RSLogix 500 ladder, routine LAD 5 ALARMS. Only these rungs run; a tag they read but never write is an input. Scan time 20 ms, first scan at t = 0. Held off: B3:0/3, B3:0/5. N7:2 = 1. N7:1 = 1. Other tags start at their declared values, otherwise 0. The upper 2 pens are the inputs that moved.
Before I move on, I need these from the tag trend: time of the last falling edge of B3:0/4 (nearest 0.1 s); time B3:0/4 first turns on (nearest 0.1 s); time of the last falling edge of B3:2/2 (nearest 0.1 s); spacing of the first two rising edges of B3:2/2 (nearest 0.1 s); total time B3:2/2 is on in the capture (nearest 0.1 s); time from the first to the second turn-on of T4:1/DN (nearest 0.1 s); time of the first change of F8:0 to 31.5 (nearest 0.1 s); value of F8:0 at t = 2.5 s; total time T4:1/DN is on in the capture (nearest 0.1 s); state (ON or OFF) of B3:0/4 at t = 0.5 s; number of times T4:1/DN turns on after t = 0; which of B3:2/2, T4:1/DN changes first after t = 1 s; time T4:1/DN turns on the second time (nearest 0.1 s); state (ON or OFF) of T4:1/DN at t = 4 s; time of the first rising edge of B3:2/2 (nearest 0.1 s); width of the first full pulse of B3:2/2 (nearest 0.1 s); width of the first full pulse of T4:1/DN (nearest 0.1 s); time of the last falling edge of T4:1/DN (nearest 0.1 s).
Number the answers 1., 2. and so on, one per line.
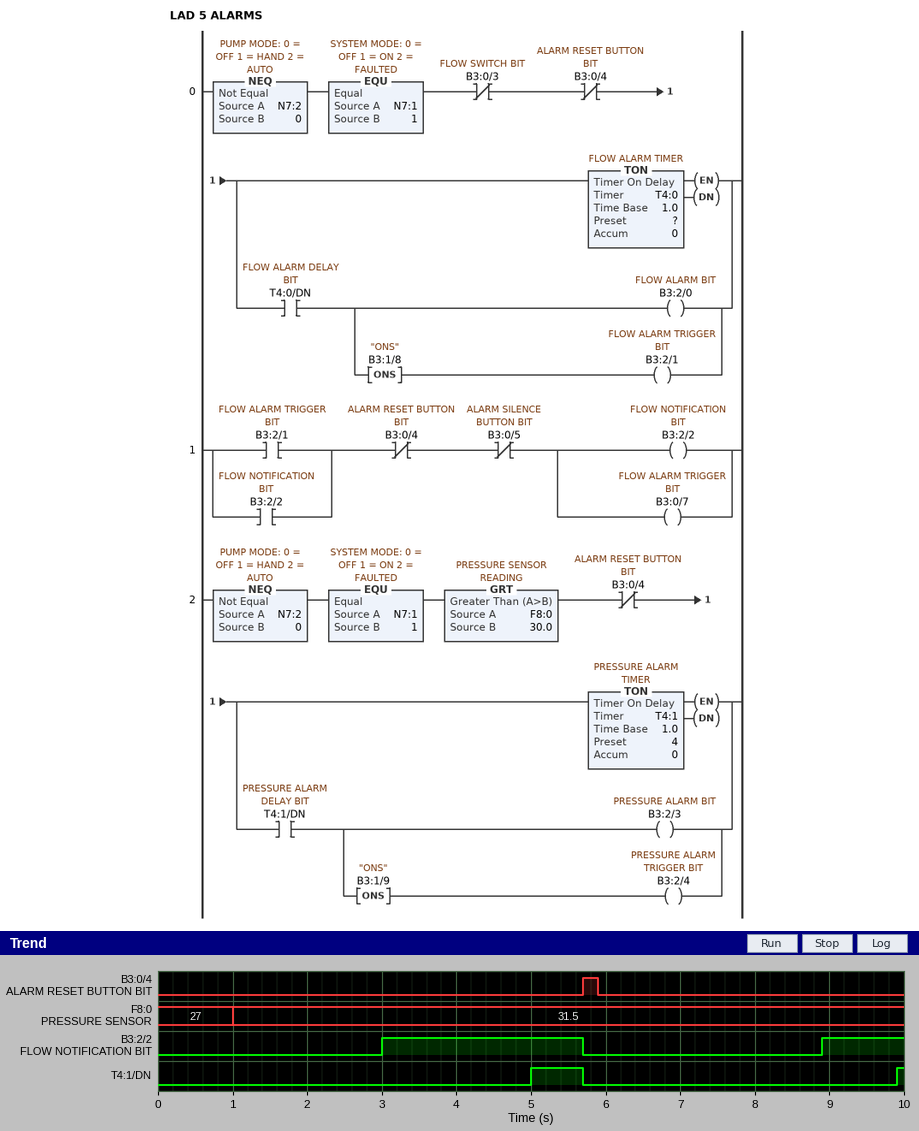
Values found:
1. 5.9 s
2. 5.7 s
3. 5.7 s
4. 5.9 s
5. 3.8 s
6. 4.9 s
7. 1.0 s
8. 31.5
9. 0.8 s
10. OFF
11. 2
12. B3:2/2
13. 9.9 s
14. OFF
15. 3.0 s
16. 2.7 s
17. 0.7 s
18. 5.7 s
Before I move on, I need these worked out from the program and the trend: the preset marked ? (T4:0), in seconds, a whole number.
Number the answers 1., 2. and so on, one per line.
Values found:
1. 3 s
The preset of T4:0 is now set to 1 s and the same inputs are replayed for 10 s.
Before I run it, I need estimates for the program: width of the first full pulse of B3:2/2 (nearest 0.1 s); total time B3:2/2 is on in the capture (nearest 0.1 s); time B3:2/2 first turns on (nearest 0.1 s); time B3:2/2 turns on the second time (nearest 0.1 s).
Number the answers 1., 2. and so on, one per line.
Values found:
1. 4.7 s
2. 7.8 s
3. 1.0 s
4. 6.9 s
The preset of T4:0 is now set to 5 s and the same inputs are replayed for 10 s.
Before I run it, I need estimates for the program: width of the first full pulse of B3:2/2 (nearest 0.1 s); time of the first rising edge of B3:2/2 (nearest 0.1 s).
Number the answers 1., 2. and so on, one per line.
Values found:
1. 0.7 s
2. 5.0 s
